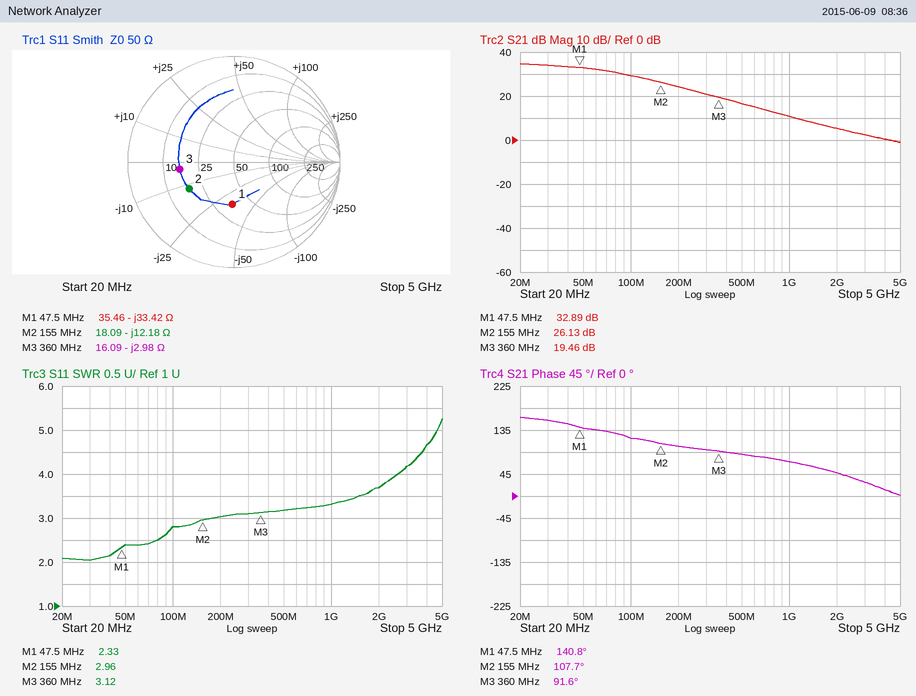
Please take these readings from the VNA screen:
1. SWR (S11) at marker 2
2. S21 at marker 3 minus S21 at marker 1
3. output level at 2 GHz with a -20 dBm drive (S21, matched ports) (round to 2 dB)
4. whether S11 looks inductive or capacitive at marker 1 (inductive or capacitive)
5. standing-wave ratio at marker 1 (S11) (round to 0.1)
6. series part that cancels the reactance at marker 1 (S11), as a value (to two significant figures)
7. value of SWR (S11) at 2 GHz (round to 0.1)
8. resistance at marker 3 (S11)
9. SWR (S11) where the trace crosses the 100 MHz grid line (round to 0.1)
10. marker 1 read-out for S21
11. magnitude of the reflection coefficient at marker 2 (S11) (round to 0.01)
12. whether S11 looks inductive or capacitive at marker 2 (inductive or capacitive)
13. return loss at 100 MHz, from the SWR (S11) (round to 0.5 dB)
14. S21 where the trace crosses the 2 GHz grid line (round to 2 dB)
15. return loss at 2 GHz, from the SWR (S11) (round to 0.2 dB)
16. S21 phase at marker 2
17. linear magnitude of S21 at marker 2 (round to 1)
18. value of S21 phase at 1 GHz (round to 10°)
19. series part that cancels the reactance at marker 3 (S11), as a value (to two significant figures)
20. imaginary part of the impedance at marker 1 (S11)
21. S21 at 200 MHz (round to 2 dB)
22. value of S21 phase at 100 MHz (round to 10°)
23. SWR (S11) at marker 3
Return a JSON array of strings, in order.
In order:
["2.96", "-13.43 dB", "-14 dBm", "capacitive", "2.3", "110 nH", "3.7", "16.09 Ω", "2.8", "32.89 dB", "0.49", "capacitive", "6.5 dB", "6 dB", "4.8 dB", "107.7°", "20", "70°", "1.3 nH", "-33.42 Ω", "24 dB", "120°", "3.12"]
